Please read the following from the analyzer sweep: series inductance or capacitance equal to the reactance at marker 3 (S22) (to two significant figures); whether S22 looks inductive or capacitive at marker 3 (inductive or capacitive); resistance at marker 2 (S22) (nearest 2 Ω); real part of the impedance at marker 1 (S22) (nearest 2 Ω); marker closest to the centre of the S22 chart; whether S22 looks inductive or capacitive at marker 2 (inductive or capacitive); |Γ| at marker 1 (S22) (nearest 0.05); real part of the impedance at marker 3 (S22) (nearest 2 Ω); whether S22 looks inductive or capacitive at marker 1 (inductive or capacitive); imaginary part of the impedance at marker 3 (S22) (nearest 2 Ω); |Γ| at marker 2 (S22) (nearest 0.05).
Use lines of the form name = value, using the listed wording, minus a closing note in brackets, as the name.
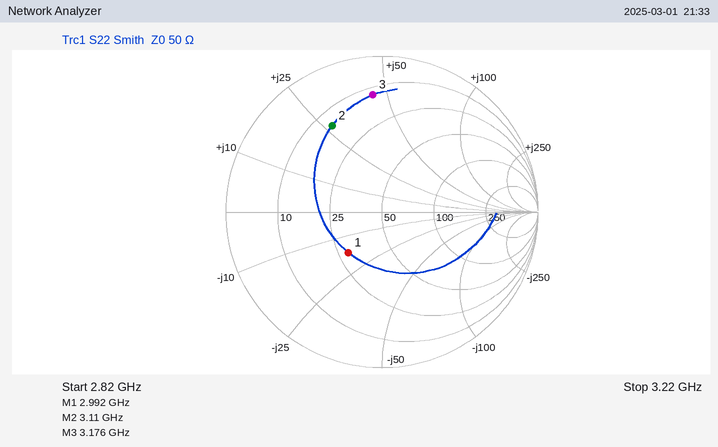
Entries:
series inductance or capacitance equal to the reactance at marker 3 (S22) = 2.2 nH
whether S22 looks inductive or capacitive at marker 3 = inductive
resistance at marker 2 (S22) = 14 Ω
real part of the impedance at marker 1 (S22) = 28 Ω
marker closest to the centre of the S22 chart = marker 1
whether S22 looks inductive or capacitive at marker 2 = inductive
|Γ| at marker 1 (S22) = 0.35
real part of the impedance at marker 3 (S22) = 12 Ω
whether S22 looks inductive or capacitive at marker 1 = capacitive
imaginary part of the impedance at marker 3 (S22) = +44 Ω
|Γ| at marker 2 (S22) = 0.65
